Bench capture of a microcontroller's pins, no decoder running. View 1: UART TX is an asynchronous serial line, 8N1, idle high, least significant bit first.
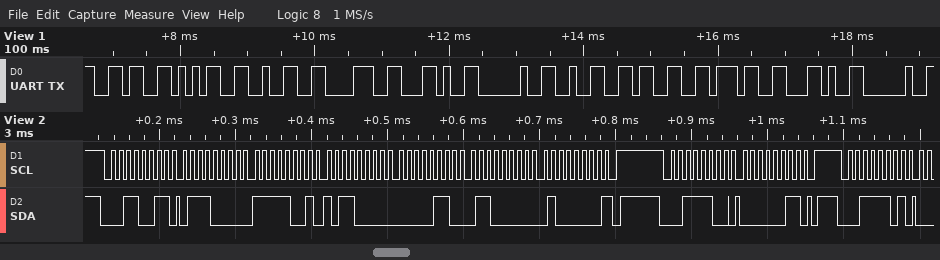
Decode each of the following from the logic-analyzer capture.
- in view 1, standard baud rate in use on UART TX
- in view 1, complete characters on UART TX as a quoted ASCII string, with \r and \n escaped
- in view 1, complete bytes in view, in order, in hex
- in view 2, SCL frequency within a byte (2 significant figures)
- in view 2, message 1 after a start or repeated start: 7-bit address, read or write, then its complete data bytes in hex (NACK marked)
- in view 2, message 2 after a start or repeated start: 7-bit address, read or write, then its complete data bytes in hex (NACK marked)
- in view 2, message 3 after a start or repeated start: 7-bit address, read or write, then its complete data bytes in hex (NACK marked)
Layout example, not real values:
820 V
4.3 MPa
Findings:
9600 baud
"6528, 237, "
36 35 32 38 2C 20 32 33 37 2C 20
100 kHz
0x19 read: 70 F9 B0 06 60 40 NACK
0x1E write: 03
0x1E read
